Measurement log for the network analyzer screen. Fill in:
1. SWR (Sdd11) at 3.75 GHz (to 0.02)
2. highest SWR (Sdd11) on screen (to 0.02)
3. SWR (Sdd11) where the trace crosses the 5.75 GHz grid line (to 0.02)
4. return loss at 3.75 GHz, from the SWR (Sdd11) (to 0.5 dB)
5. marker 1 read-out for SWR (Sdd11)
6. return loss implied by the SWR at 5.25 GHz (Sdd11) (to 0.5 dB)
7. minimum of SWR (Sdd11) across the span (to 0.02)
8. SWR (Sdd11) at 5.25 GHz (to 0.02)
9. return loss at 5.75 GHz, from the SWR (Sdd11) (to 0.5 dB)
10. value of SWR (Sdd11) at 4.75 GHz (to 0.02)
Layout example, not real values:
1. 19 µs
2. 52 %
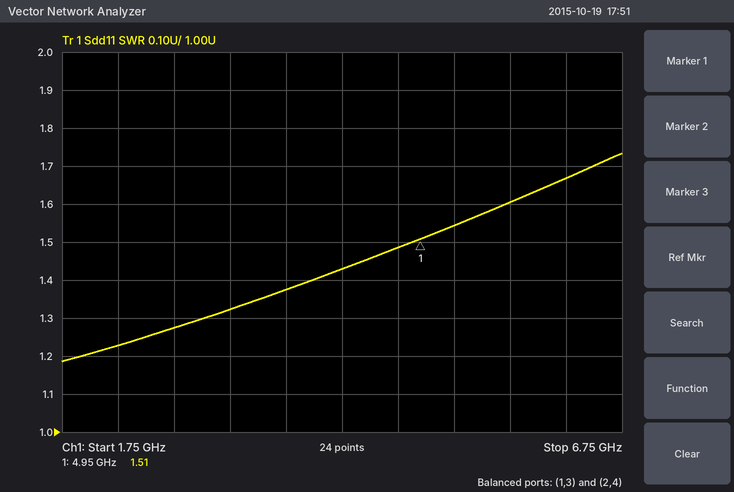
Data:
1. 1.38
2. 1.74
3. 1.60
4. 16.0 dB
5. 1.51
6. 13.5 dB
7. 1.18
8. 1.54
9. 12.5 dB
10. 1.48
